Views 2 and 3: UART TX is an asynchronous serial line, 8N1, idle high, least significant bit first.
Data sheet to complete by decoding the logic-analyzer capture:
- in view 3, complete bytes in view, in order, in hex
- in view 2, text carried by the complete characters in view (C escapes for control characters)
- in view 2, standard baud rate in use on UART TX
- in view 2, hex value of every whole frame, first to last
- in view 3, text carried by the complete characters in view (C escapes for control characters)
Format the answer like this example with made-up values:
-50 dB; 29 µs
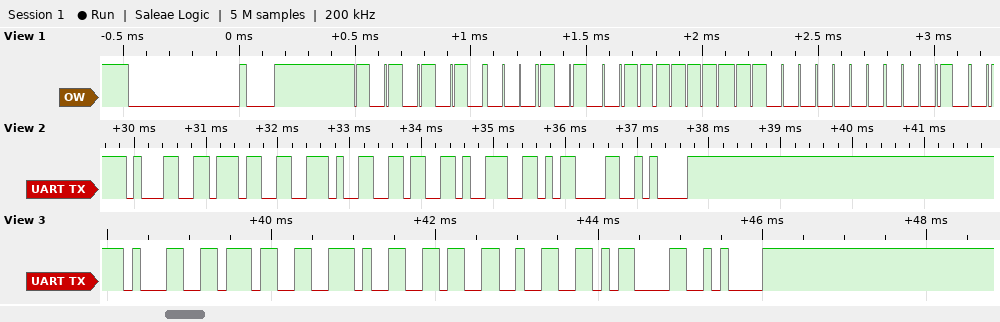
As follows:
31 37 2E 36 32 0D 0A; "17.69\r\n"; 9600 baud; 0x31 0x37 0x2E 0x36 0x39 0x0D 0x0A; "17.62\r\n"
